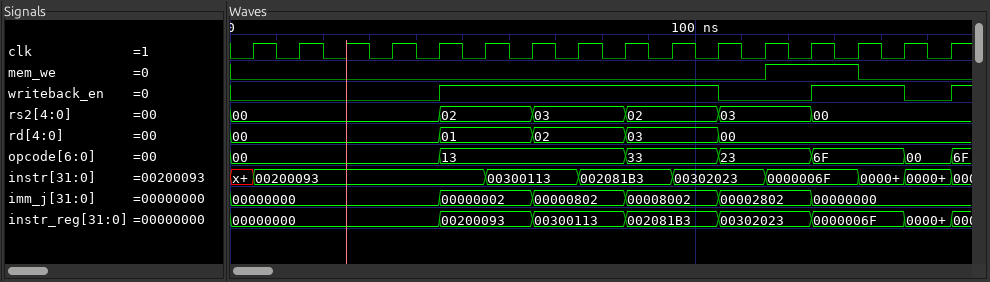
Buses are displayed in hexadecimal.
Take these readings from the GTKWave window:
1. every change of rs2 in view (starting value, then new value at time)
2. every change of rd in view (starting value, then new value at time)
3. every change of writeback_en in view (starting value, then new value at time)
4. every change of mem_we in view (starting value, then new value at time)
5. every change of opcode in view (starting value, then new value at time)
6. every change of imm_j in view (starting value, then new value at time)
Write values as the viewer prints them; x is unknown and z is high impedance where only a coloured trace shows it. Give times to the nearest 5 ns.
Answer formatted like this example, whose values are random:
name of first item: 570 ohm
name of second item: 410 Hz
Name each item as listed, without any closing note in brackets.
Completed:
every change of rs2 in view: 00, 02 at 45 ns, 03 at 65 ns, 02 at 85 ns, 03 at 105 ns, 00 at 125 ns
every change of rd in view: 00, 01 at 45 ns, 02 at 65 ns, 03 at 85 ns, 00 at 105 ns
every change of writeback_en in view: 0, 1 at 45 ns, 0 at 105 ns, 1 at 125 ns, 0 at 145 ns, 1 at 155 ns
every change of mem_we in view: 0, 1 at 115 ns, 0 at 135 ns
every change of opcode in view: 00, 13 at 45 ns, 33 at 85 ns, 23 at 105 ns, 6F at 125 ns, 00 at 145 ns, 6F at 155 ns
every change of imm_j in view: 00000000, 00000002 at 45 ns, 00000802 at 65 ns, 00008002 at 85 ns, 00002802 at 105 ns, 00000000 at 125 ns
